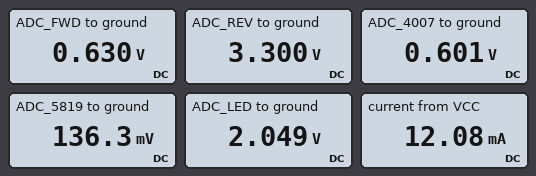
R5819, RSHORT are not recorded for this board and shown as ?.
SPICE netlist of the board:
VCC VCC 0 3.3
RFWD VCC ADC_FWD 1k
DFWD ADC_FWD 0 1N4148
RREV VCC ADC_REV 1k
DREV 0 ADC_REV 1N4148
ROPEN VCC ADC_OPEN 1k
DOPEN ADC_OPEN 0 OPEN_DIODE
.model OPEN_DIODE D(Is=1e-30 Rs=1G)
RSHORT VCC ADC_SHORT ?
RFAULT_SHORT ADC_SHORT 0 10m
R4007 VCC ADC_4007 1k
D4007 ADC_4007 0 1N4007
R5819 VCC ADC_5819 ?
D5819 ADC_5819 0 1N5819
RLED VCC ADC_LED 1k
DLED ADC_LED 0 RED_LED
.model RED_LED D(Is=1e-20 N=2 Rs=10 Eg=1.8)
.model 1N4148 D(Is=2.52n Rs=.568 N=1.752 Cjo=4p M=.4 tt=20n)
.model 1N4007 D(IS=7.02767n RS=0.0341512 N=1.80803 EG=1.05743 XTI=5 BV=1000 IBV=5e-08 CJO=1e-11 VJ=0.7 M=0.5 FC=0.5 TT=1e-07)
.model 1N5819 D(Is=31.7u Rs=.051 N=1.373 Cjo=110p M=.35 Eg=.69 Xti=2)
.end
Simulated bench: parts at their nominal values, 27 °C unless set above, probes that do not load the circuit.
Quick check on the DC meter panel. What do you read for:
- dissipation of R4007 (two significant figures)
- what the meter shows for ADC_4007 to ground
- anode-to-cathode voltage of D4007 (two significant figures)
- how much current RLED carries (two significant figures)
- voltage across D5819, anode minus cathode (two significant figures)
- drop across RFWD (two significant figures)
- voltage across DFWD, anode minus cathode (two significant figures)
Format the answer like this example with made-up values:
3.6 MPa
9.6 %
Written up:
7.3 mW
0.601 V
600 mV
1.3 mA
140 mV
2.7 V
630 mV
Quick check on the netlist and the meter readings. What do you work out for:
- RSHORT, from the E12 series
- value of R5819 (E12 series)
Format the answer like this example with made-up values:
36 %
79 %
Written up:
820 Ω
2.2 kΩ
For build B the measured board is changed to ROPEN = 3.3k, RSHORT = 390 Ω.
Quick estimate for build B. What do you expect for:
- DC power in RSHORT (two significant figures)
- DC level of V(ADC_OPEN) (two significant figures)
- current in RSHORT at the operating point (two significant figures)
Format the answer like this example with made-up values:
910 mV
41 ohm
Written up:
28 mW
3.3 V
8.5 mA
